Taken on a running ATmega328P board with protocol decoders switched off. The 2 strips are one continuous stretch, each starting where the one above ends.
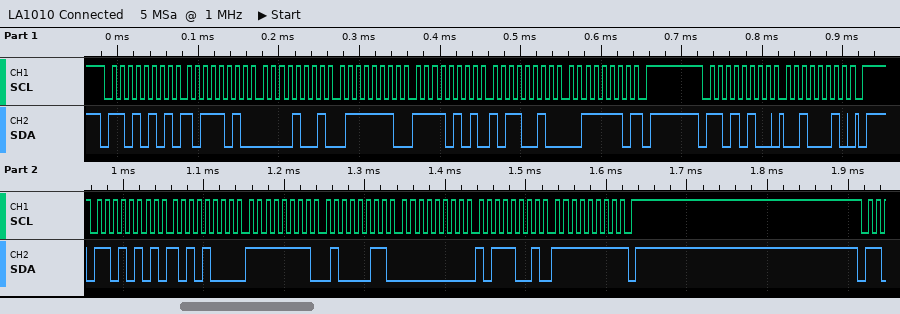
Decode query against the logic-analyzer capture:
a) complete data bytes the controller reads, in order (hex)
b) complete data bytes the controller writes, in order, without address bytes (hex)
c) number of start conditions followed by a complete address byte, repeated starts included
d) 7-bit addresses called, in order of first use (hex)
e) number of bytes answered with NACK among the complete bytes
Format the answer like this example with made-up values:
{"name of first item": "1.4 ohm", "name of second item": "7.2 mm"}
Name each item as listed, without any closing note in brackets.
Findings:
{"complete data bytes the controller reads, in order": "BA 09 7E F5 B2 3E A8 FF 43 00 B9 FF", "complete data bytes the controller writes, in order, without address bytes": "22", "number of start conditions followed by a complete address byte, repeated starts included": "3", "7-bit addresses called, in order of first use": "0x6A", "number of bytes answered with NACK among the complete bytes": "2"}
